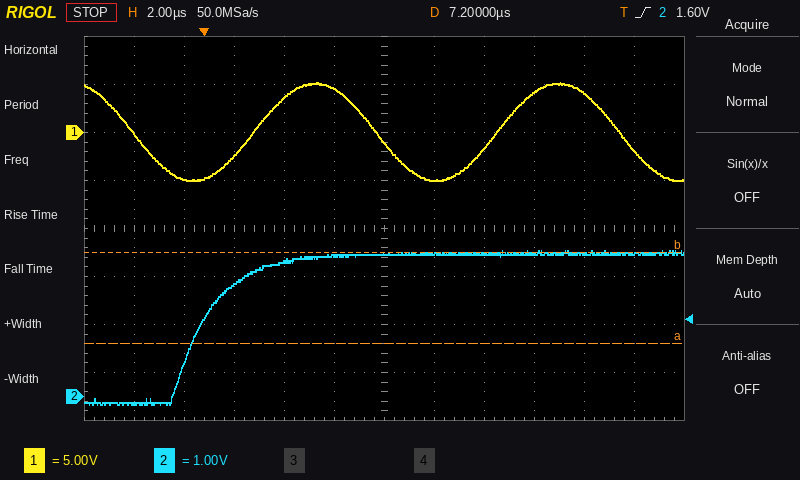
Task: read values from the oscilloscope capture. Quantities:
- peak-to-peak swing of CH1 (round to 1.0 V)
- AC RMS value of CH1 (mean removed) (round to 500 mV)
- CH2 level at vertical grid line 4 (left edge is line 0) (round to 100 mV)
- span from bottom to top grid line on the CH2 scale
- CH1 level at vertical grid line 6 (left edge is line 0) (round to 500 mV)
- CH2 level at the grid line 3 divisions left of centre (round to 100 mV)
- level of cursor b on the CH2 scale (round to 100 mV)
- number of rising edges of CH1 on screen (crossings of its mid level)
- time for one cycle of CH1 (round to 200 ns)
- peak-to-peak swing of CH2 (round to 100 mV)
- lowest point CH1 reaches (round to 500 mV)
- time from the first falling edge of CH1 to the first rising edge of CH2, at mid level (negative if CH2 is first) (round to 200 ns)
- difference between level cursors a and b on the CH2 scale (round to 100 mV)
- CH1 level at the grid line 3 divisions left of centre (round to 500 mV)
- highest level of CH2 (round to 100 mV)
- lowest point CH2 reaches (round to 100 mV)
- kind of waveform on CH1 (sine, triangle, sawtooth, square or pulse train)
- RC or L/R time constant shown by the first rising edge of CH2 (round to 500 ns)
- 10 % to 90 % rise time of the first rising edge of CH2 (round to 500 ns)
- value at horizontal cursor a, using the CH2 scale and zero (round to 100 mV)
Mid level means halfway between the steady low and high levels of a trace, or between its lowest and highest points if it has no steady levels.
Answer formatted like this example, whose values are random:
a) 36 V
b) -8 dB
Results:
a) 10.0 V
b) 3.5 V
c) 2.8 V
d) 8 V
e) -1.0 V
f) 2.3 V
g) 3.0 V
h) 2
i) 9.8 µs
j) 3.2 V
k) -5.0 V
l) +2.6 µs
m) 1.9 V
n) -2.5 V
o) 3.0 V
p) -200 mV
q) sine
r) 1.5 µs
s) 3.5 µs
t) 1.1 V
